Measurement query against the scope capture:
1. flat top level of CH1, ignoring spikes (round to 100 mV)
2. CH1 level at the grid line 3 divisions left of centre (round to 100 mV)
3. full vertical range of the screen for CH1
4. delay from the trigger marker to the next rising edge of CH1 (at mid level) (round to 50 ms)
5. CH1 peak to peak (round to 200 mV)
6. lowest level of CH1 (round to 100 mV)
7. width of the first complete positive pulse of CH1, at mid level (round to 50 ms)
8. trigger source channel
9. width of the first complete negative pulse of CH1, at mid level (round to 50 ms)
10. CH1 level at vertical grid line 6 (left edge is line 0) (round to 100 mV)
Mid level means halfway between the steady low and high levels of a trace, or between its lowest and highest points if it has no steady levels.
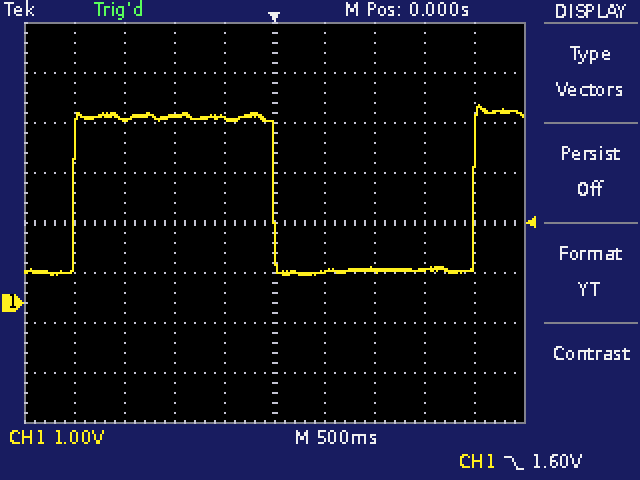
3.7 V
3.7 V
8 V
2.00 s
3.4 V
600 mV
2.00 s
CH1
2.00 s
600 mV
